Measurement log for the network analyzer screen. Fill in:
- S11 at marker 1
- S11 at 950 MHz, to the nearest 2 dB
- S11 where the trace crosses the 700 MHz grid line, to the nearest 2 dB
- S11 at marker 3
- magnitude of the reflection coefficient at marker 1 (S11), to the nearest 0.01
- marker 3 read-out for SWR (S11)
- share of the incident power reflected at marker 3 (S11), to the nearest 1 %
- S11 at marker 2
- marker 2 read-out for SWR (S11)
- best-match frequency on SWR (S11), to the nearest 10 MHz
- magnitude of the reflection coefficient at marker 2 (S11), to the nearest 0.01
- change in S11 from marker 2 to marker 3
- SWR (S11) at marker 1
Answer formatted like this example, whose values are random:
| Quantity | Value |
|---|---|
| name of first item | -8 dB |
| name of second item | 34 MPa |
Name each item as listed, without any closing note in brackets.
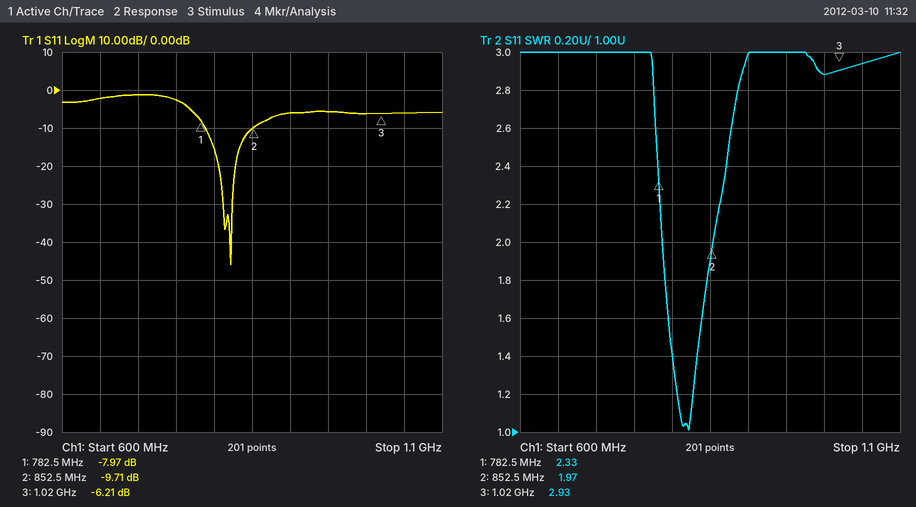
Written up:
| Quantity | Value |
|---|---|
| S11 at marker 1 | -7.97 dB |
| S11 at 950 MHz, to the nearest 2 dB | -6 dB |
| S11 where the trace crosses the 700 MHz grid line, to the nearest 2 dB | -2 dB |
| S11 at marker 3 | -6.21 dB |
| magnitude of the reflection coefficient at marker 1 (S11), to the nearest 0.01 | 0.40 |
| marker 3 read-out for SWR | 2.93 |
| share of the incident power reflected at marker 3 (S11), to the nearest 1 % | 24 % |
| S11 at marker 2 | -9.71 dB |
| marker 2 read-out for SWR | 1.97 |
| best-match frequency on SWR (S11), to the nearest 10 MHz | 820 MHz |
| magnitude of the reflection coefficient at marker 2 (S11), to the nearest 0.01 | 0.33 |
| change in S11 from marker 2 to marker 3 | 3.50 dB |
| SWR (S11) at marker 1 | 2.33 |
